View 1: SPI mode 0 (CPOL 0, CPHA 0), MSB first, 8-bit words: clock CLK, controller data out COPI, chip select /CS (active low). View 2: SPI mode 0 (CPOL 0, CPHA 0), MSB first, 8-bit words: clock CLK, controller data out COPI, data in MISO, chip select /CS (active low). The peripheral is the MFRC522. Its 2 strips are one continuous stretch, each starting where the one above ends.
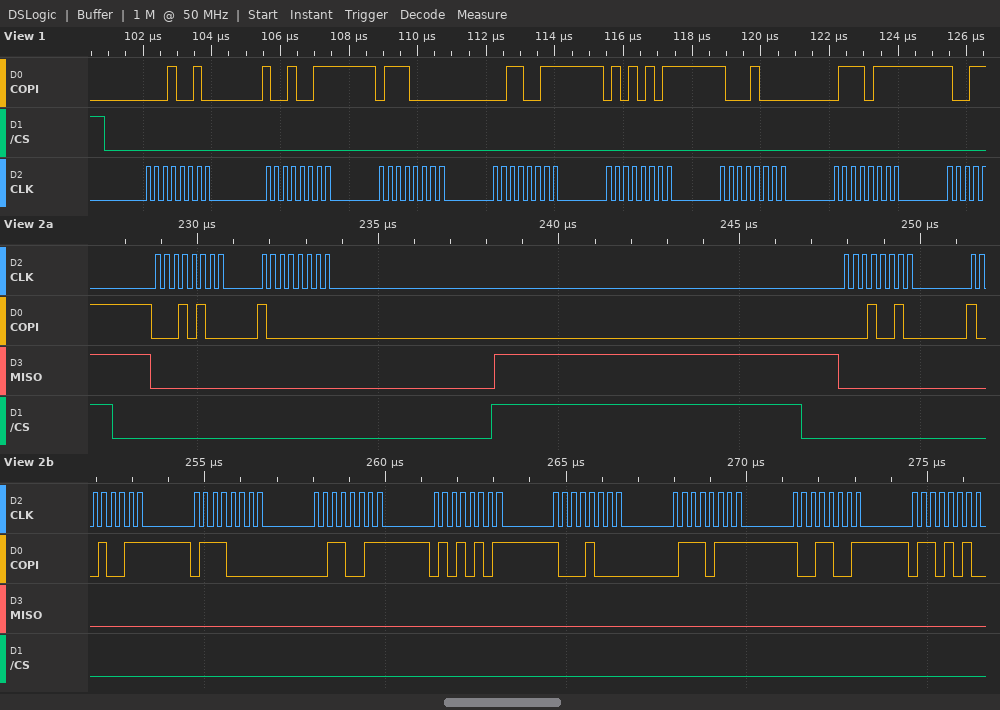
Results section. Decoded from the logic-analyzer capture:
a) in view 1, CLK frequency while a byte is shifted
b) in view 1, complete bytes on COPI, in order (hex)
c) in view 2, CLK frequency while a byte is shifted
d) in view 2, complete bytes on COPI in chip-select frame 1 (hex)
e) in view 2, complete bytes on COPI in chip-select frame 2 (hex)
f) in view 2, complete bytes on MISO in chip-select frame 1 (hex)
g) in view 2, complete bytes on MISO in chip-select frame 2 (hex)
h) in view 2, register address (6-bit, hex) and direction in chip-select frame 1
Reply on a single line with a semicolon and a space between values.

4 MHz; 12 93 70 33 55 88 77; 4 MHz; 0x14 0x80; 0x12 0x93 0x70 0x33 0x55 0x88 0x77 0x99 0x6A; 0x00 0x00; 0x00 0x00 0x00 0x00 0x00 0x00 0x00 0x00 0x00; 0x0A write
